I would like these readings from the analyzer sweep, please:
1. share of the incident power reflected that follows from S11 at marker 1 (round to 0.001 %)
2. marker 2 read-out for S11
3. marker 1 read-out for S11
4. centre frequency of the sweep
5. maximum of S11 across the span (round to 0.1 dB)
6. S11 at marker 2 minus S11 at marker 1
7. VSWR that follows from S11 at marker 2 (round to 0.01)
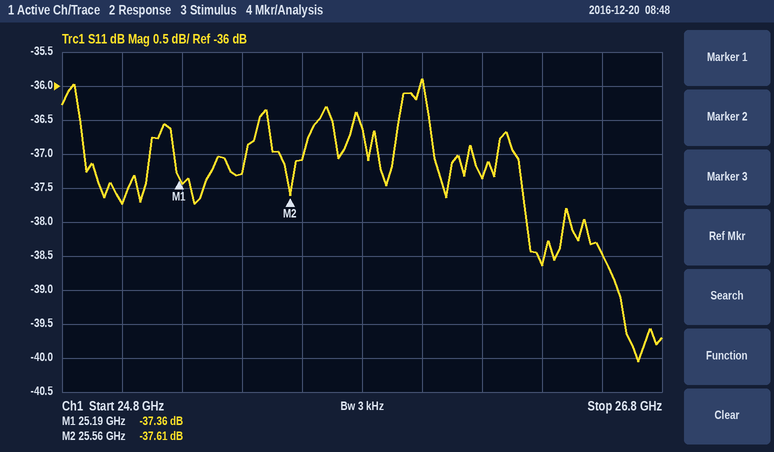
0.018 %
-37.61 dB
-37.36 dB
25.8 GHz
-35.9 dB
-0.25 dB
1.03
